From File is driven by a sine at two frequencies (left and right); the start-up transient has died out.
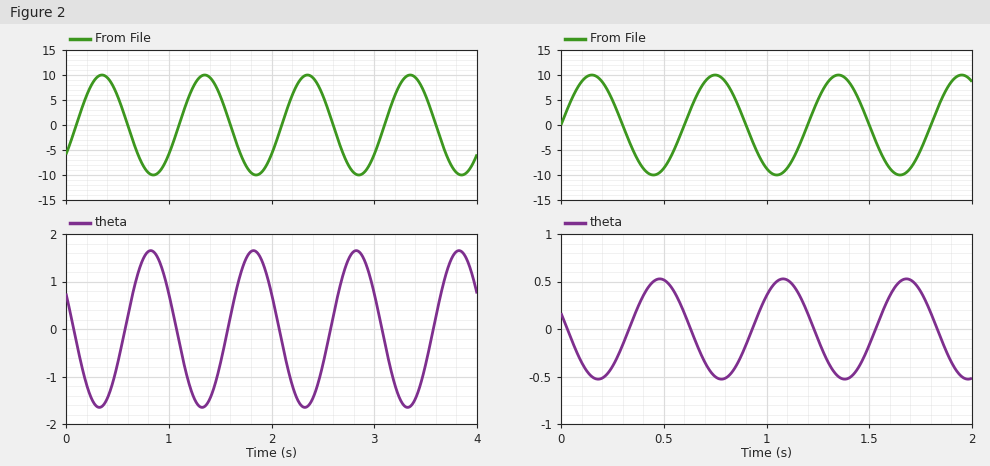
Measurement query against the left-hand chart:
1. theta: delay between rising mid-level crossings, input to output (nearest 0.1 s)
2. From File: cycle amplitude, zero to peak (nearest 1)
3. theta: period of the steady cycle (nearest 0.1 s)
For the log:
0.5 s
10
1.0 s
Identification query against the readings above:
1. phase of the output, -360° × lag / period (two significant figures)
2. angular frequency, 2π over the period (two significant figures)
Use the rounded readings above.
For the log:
-180°
6.3 rad/s
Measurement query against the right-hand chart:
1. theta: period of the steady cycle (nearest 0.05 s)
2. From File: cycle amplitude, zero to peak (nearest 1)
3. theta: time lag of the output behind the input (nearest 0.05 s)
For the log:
0.60 s
10
0.35 s
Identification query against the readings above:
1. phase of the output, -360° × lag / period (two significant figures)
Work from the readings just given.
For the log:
-210°
